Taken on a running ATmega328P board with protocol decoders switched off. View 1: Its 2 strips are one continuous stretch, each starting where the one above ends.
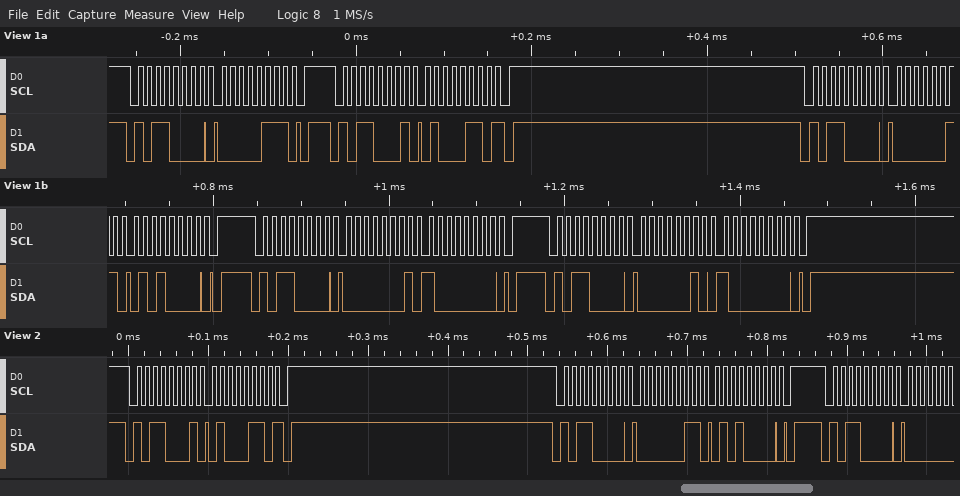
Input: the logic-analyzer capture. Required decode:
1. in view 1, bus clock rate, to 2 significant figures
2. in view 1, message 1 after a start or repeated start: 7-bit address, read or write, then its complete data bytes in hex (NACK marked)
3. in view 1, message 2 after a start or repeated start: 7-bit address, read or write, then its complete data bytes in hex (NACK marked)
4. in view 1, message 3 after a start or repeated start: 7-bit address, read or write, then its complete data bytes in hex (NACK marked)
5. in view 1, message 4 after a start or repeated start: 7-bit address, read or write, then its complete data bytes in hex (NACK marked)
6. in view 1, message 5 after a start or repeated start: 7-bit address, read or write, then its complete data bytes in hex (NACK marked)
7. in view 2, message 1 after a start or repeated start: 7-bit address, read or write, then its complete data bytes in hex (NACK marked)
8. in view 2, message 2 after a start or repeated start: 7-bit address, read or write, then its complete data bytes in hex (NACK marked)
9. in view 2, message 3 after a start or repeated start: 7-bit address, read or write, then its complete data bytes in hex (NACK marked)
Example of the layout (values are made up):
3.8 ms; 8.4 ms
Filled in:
100 kHz; 0x58 write: 07; 0x58 read: 46 NACK; 0x58 write: 03 50; 0x58 write: 01 80; 0x58 write: 02 80; 0x58 read: 46 NACK; 0x58 write: 03 50; 0x58 write
